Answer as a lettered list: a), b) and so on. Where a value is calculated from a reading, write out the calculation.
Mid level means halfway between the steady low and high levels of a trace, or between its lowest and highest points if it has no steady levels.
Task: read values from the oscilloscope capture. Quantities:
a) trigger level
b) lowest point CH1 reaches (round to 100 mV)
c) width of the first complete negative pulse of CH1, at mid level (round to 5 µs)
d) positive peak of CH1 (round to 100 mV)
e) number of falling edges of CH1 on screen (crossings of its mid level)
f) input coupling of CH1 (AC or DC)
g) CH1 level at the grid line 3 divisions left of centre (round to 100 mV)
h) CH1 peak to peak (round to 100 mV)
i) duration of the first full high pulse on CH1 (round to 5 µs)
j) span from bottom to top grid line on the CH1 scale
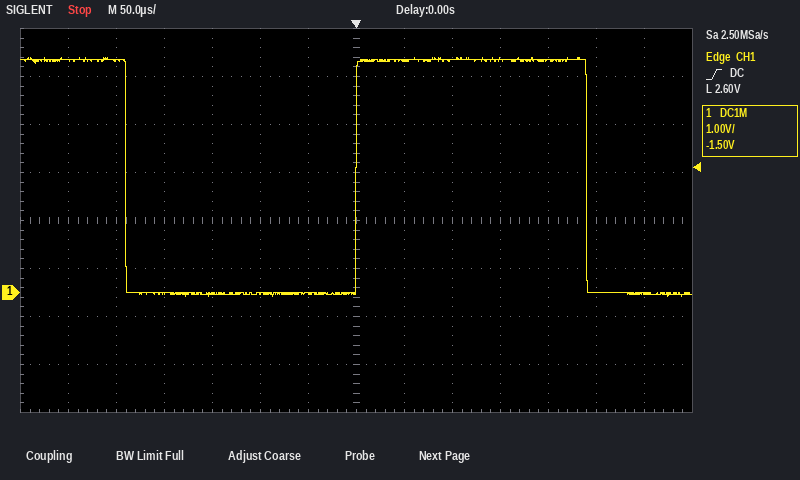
a) 2.60 V
b) -100 mV
c) 240 µs
d) 4.9 V
e) 2
f) DC
g) 0.0 V
h) 4.9 V − (-100 mV) = 5.0 V
i) 240 µs
j) 8 V
